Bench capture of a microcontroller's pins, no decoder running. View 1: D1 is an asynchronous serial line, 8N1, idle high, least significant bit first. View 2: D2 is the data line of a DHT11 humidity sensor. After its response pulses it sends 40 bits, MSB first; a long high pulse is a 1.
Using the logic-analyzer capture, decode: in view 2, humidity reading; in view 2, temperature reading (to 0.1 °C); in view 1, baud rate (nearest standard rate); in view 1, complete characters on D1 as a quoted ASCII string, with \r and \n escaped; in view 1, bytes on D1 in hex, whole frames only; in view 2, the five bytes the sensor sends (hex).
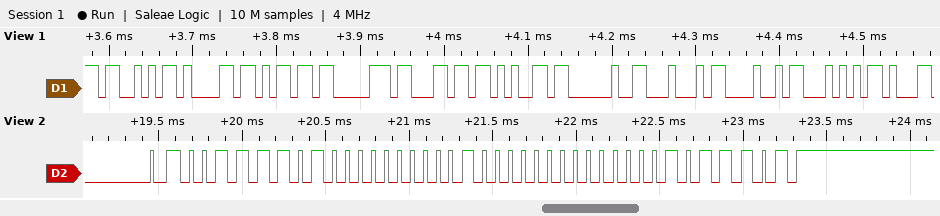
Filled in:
61 %
32.0 °C
115200 baud
"Sample DHT"
0x53 0x61 0x6D 0x70 0x6C 0x65 0x20 0x44 0x48 0x54
3D 00 20 00 5D
